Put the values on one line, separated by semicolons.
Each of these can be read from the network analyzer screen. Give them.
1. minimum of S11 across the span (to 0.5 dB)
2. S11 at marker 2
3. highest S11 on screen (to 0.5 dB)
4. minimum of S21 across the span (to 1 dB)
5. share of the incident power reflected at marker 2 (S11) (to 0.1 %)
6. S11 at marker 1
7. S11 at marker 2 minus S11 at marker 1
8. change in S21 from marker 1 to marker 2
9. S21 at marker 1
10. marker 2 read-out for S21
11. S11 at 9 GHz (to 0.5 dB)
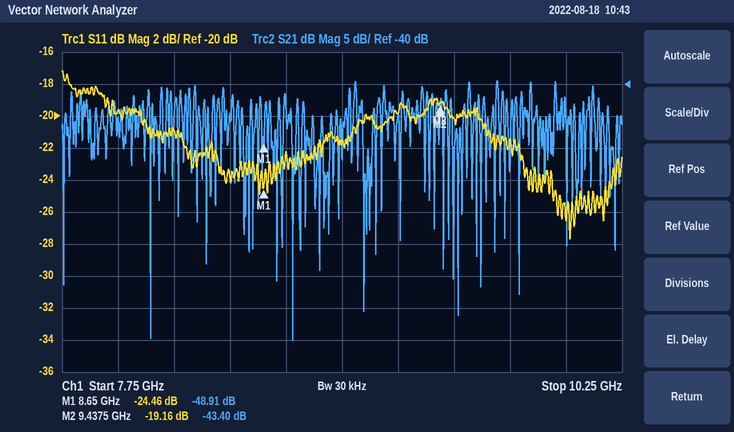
-27.5 dB; -19.16 dB; -17.0 dB; -80 dB; 1.2 %; -24.46 dB; 5.30 dB; 5.51 dB; -48.91 dB; -43.40 dB; -21.5 dB
